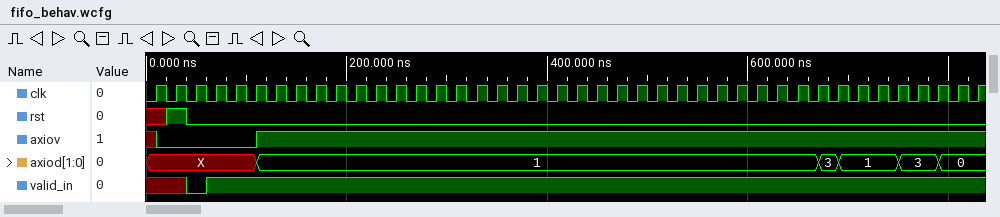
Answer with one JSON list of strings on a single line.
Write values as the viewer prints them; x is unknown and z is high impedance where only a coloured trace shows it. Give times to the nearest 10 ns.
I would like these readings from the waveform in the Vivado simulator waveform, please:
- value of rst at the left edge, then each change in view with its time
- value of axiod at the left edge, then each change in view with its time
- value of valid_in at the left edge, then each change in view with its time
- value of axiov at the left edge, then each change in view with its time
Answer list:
["x, 1 at 20 ns, 0 at 40 ns", "X, 1 at 110 ns, 3 at 670 ns, 1 at 690 ns, 3 at 750 ns, 0 at 790 ns", "x, 0 at 40 ns, 1 at 60 ns", "x, 0 at 10 ns, 1 at 110 ns"]
